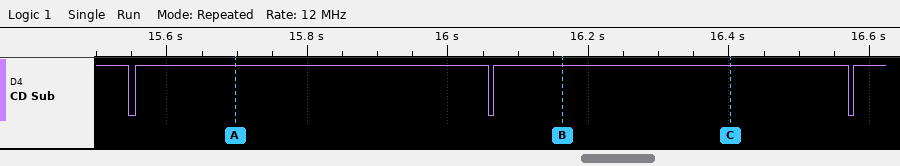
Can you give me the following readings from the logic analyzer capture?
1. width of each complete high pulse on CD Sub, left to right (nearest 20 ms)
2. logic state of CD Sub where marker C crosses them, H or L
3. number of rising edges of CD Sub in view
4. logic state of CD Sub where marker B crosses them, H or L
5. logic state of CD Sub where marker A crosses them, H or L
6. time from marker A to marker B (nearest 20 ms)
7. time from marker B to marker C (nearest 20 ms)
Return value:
500 ms, 500 ms
CD Sub=H
3
CD Sub=H
CD Sub=H
460 ms
240 ms
